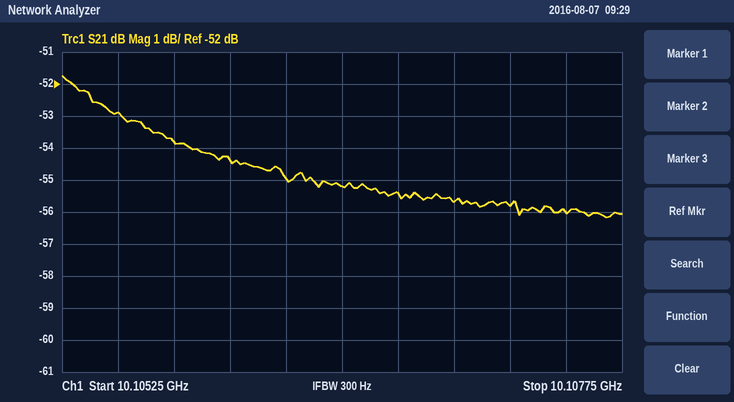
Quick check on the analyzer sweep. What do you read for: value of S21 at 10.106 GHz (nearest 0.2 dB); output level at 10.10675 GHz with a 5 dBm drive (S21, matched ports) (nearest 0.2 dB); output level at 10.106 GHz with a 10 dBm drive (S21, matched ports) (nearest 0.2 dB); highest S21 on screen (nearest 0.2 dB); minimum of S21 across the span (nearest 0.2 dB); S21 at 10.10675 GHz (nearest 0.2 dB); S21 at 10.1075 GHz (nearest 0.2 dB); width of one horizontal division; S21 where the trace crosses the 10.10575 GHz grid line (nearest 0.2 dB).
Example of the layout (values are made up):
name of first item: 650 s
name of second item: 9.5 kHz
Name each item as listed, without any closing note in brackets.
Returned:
value of S21 at 10.106 GHz: -54.4 dB
output level at 10.10675 GHz with a 5 dBm drive (S21, matched ports): -50.4 dBm
output level at 10.106 GHz with a 10 dBm drive (S21, matched ports): -44.4 dBm
highest S21 on screen: -51.8 dB
minimum of S21 across the span: -56.2 dB
S21 at 10.10675 GHz: -55.4 dB
S21 at 10.1075 GHz: -56.0 dB
width of one horizontal division: 250 kHz
S21 where the trace crosses the 10.10575 GHz grid line: -53.8 dB
